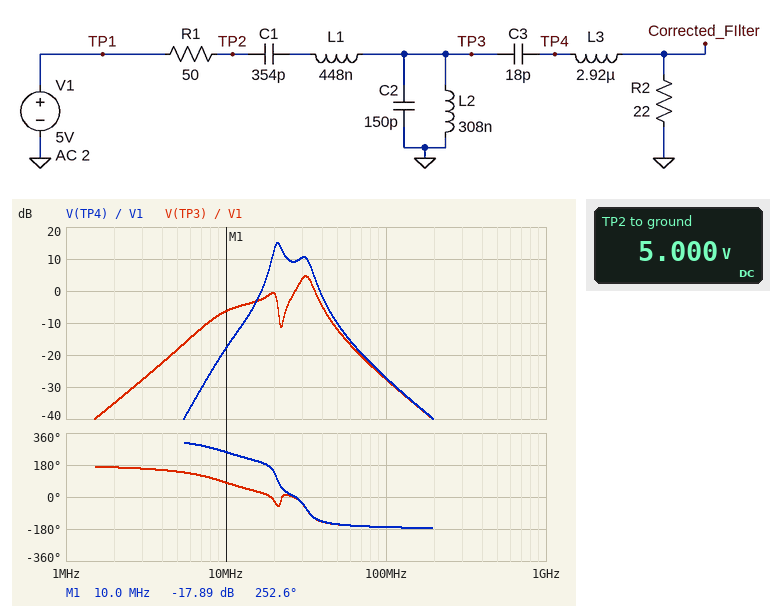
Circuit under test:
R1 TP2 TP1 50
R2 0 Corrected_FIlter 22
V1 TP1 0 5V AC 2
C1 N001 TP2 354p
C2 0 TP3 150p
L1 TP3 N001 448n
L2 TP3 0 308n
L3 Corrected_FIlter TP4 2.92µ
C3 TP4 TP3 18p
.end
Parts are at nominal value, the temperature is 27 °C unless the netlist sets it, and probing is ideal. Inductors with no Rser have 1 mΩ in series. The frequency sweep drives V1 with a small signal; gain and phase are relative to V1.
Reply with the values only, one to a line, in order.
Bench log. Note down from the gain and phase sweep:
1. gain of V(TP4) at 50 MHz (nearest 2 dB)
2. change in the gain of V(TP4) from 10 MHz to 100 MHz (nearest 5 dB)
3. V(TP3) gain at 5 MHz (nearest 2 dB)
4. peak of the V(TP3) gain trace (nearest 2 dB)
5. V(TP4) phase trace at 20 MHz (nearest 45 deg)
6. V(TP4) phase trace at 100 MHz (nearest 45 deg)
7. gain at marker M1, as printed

-10 dB
-10 dB
-18 dB
4 dB
135 deg
-180 deg
-17.89 dB
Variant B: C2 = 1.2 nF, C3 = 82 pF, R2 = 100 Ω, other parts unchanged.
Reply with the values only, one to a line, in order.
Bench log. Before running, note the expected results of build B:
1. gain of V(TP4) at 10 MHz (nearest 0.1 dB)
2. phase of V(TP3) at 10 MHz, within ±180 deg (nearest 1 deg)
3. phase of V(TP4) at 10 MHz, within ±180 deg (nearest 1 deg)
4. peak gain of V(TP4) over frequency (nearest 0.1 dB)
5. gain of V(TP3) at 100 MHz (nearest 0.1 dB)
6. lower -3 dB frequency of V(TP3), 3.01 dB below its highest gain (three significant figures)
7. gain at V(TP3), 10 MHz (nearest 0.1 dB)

-0.5 dB
-29 deg
38 deg
0.2 dB
-46.4 dB
6.52 MHz
-6.8 dB
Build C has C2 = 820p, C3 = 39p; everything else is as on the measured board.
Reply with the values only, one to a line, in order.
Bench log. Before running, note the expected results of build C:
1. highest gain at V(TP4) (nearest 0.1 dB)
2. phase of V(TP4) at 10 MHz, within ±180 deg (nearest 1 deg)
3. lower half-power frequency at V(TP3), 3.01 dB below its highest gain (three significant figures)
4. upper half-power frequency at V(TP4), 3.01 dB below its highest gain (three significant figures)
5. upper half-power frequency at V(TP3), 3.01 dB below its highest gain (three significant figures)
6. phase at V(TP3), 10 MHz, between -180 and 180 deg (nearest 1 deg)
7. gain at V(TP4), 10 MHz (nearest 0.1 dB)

11.8 dB
157 deg
7.66 MHz
16.3 MHz
10.6 MHz
-11 deg
-2.7 dB
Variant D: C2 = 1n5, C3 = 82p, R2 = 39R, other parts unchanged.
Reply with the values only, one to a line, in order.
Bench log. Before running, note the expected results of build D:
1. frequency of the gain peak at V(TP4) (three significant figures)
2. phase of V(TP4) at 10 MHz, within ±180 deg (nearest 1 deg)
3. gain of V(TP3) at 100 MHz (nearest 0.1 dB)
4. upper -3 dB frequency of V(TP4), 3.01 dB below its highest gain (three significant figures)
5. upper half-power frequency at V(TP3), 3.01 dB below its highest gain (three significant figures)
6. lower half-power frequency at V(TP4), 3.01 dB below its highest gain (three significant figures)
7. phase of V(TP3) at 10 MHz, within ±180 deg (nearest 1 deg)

10.7 MHz
59 deg
-48.4 dB
11.8 MHz
7.11 MHz
9.46 MHz
-34 deg
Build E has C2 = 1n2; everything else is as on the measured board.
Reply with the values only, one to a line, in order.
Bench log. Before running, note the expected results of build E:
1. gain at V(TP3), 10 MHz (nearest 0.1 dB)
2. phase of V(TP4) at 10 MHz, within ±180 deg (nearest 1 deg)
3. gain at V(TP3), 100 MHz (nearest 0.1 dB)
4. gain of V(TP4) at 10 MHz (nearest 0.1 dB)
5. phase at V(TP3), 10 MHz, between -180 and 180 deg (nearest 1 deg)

-5.6 dB
130 deg
-46.4 dB
-17.2 dB
-41 deg
